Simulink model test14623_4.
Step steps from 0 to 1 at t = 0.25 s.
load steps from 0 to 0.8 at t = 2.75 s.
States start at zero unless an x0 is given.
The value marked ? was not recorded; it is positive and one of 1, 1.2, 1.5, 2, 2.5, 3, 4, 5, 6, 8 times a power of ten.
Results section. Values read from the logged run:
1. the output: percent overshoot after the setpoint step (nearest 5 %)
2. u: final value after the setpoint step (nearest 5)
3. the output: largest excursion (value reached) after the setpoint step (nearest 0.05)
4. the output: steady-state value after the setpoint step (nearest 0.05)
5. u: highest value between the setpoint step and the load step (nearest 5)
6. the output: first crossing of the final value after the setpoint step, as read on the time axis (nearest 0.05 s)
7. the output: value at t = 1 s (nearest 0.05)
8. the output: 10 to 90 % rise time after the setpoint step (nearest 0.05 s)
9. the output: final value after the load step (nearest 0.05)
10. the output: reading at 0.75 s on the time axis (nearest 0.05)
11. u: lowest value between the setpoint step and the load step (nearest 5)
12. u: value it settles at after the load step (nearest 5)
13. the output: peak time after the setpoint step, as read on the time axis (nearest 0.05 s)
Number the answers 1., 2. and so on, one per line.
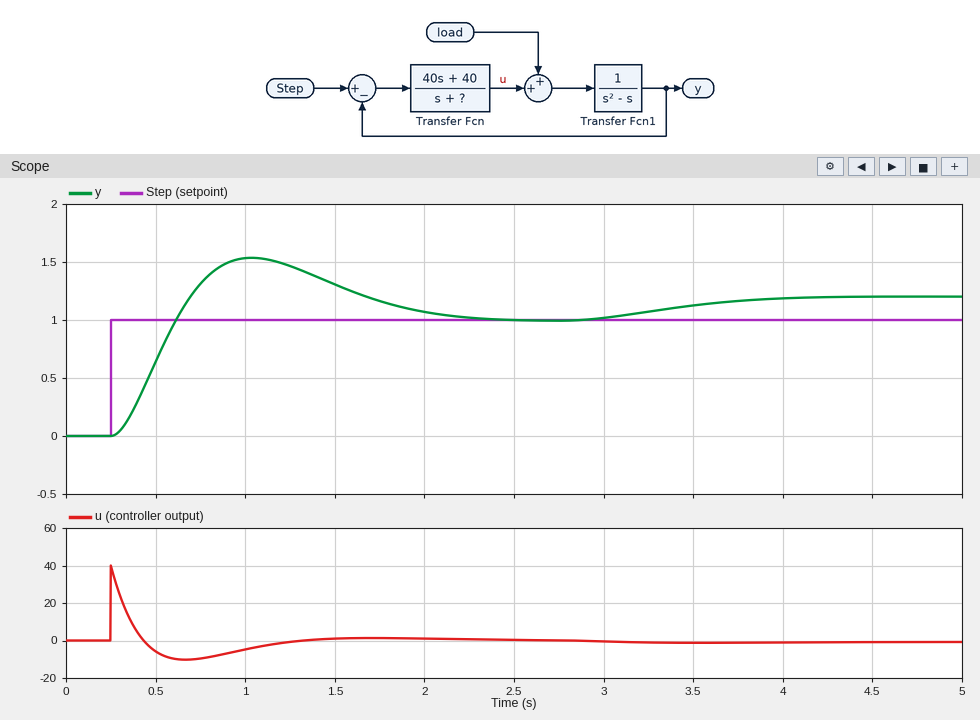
1. 55 %
2. 0
3. 1.55
4. 1.00
5. 40
6. 0.60 s
7. 1.55
8. 0.25 s
9. 1.20
10. 1.30
11. -10
12. 0
13. 1.05 s
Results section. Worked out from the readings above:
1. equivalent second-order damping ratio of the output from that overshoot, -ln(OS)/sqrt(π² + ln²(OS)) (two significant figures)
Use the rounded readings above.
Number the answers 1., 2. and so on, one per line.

1. 0.19
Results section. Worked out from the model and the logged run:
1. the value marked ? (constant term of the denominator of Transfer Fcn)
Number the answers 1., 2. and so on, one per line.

1. 10
